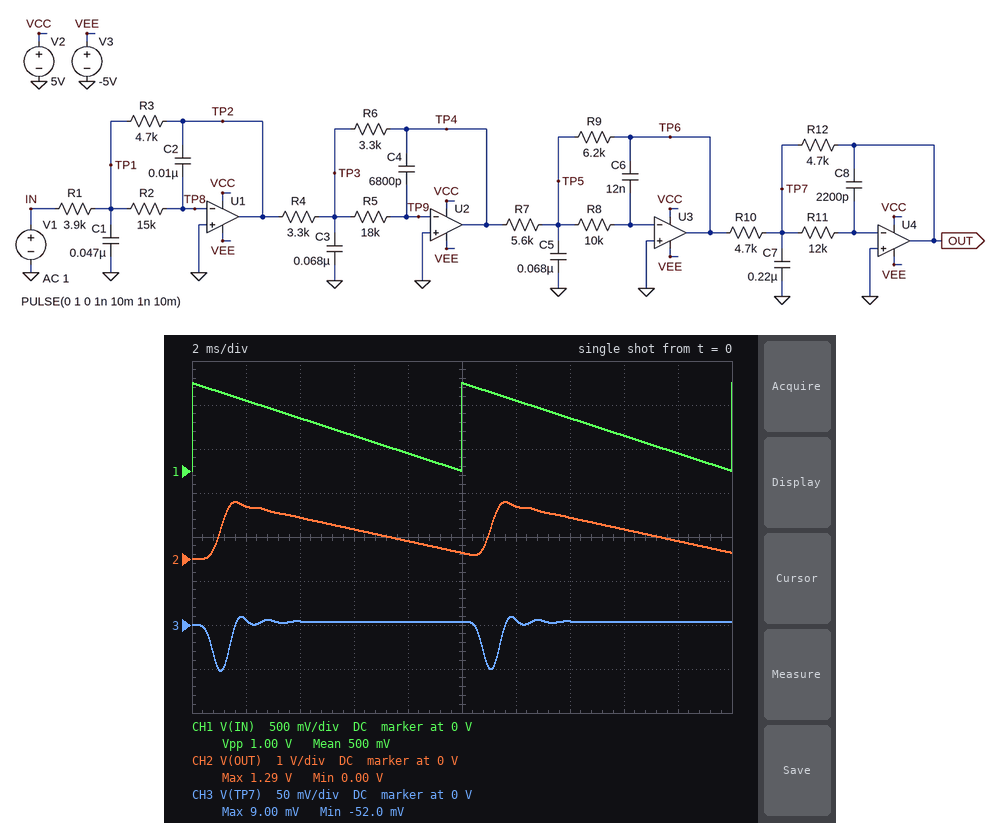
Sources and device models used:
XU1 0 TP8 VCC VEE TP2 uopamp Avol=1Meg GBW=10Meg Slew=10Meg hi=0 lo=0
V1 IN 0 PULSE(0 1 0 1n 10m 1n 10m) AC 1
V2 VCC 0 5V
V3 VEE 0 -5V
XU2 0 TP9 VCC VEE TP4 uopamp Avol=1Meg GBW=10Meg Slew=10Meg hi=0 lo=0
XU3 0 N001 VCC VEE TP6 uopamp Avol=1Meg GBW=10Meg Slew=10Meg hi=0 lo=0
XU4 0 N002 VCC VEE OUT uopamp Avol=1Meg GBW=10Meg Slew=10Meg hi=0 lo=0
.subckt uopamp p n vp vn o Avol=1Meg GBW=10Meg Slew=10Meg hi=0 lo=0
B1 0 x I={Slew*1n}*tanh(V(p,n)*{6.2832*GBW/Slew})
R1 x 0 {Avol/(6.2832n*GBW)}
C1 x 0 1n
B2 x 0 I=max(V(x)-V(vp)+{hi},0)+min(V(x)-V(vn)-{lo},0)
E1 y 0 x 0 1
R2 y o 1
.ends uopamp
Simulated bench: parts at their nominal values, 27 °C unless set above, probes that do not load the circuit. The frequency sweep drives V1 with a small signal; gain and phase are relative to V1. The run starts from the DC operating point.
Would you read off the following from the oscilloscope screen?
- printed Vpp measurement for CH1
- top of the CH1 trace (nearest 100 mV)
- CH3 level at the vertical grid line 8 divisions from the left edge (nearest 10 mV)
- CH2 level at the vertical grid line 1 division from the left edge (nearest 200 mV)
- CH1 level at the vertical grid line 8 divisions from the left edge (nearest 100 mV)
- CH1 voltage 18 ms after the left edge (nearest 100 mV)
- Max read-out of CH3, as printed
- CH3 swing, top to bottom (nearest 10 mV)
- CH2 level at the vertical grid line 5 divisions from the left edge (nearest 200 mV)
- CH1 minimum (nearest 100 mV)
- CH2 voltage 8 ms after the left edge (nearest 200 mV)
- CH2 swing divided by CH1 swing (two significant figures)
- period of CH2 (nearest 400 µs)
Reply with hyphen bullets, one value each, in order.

- 1.00 V
- 1.0 V
- 0 V
- 1.2 V
- 400 mV
- 200 mV
- 9.00 mV
- 60 mV
- 200 mV
- 0 V
- 400 mV
- 1.3
- 10.0 ms
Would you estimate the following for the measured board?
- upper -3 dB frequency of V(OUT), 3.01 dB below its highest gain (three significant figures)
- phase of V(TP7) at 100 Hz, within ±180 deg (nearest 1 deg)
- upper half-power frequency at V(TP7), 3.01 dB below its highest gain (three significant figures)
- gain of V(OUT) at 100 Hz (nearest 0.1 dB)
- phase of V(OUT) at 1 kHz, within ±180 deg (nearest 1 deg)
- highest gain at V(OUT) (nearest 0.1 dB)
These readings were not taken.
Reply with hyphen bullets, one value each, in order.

- 561 Hz
- -127 deg
- 981 Hz
- 2.4 dB
- -47 deg
- 2.5 dB
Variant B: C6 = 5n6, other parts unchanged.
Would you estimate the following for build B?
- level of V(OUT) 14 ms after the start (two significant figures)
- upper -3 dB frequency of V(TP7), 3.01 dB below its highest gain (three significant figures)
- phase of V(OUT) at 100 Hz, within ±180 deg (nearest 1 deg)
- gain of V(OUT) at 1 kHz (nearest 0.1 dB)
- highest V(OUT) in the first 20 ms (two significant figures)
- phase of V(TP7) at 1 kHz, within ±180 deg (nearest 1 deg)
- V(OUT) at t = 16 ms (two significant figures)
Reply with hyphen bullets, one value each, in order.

- 910 mV
- 1.02 kHz
- -31 deg
- -1.4 dB
- 1.5 V
- -107 deg
- 650 mV
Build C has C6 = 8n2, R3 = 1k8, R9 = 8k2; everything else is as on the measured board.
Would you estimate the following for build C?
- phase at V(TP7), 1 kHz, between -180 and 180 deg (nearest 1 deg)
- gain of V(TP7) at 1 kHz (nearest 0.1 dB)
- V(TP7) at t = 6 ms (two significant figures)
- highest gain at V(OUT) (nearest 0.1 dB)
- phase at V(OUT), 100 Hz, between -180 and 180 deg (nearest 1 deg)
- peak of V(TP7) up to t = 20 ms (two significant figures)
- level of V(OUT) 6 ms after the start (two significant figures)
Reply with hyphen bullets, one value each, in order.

- -111 deg
- -25.0 dB
- 1.8 mV
- -3.1 dB
- -30 deg
- 13 mV
- 330 mV
